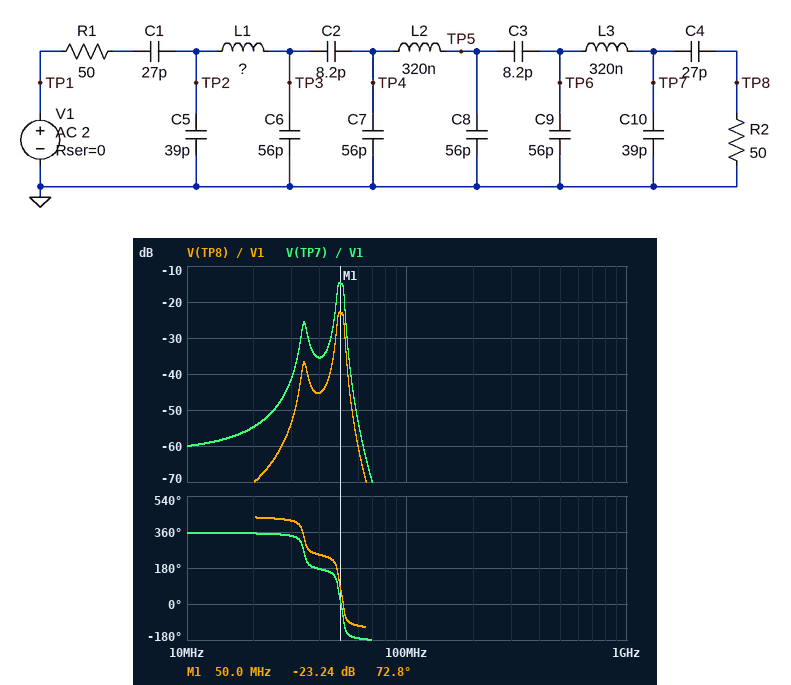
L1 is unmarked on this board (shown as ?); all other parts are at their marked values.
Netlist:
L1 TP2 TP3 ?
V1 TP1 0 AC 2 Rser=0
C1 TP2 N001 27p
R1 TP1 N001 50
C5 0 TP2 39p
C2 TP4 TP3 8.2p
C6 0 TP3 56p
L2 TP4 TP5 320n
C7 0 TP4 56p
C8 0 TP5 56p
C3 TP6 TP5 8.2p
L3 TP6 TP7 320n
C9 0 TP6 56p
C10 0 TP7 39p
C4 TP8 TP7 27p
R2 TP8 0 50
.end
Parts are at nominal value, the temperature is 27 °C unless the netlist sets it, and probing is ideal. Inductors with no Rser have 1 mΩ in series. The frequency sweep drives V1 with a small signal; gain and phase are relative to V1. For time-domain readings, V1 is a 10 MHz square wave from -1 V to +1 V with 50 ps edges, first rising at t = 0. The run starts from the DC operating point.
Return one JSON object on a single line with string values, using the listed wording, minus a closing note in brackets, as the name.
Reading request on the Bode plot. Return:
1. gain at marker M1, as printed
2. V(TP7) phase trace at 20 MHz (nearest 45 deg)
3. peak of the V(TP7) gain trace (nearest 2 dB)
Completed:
{"gain at marker M1, as printed": "-23.24 dB", "V(TP7) phase trace at 20 MHz": "360 deg", "peak of the V(TP7) gain trace": "-14 dB"}
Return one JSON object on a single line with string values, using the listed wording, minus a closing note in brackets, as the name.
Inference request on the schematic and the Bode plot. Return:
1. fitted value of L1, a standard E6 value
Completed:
{"fitted value of L1, a standard E6 value": "680 nH"}
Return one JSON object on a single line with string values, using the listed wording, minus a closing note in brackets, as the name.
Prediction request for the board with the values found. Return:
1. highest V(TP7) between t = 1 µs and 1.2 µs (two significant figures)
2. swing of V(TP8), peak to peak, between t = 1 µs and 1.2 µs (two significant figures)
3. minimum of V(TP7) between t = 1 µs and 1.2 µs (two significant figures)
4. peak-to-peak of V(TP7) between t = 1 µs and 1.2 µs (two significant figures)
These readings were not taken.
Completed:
{"highest V(TP7) between t = 1 µs and 1.2 µs": "50 mV", "swing of V(TP8), peak to peak, between t = 1 µs and 1.2 µs": "37 mV", "minimum of V(TP7) between t = 1 µs and 1.2 µs": "-48 mV", "peak-to-peak of V(TP7) between t = 1 µs and 1.2 µs": "98 mV"}
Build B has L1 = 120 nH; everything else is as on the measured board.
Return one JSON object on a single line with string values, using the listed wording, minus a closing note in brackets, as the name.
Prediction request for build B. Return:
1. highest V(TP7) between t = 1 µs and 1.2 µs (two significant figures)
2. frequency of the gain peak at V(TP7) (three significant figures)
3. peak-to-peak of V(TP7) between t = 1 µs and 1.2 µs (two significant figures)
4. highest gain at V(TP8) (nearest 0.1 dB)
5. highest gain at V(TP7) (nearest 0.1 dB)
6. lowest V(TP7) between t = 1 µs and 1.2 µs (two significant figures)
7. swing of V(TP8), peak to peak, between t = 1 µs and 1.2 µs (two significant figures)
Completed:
{"highest V(TP7) between t = 1 µs and 1.2 µs": "82 mV", "frequency of the gain peak at V(TP7)": "49.1 MHz", "peak-to-peak of V(TP7) between t = 1 µs and 1.2 µs": "160 mV", "highest gain at V(TP8)": "-18.0 dB", "highest gain at V(TP7)": "-9.7 dB", "lowest V(TP7) between t = 1 µs and 1.2 µs": "-80 mV", "swing of V(TP8), peak to peak, between t = 1 µs and 1.2 µs": "63 mV"}
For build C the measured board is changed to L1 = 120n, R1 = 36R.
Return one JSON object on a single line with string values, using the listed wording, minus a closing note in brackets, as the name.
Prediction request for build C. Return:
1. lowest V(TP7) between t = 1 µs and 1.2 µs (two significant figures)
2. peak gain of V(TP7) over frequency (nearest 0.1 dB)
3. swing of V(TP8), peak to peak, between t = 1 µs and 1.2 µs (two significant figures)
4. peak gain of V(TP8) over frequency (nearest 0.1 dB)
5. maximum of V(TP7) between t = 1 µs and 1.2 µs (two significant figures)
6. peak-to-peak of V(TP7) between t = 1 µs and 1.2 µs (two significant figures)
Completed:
{"lowest V(TP7) between t = 1 µs and 1.2 µs": "-83 mV", "peak gain of V(TP7) over frequency": "-9.4 dB", "swing of V(TP8), peak to peak, between t = 1 µs and 1.2 µs": "65 mV", "peak gain of V(TP8) over frequency": "-17.7 dB", "maximum of V(TP7) between t = 1 µs and 1.2 µs": "85 mV", "peak-to-peak of V(TP7) between t = 1 µs and 1.2 µs": "170 mV"}
